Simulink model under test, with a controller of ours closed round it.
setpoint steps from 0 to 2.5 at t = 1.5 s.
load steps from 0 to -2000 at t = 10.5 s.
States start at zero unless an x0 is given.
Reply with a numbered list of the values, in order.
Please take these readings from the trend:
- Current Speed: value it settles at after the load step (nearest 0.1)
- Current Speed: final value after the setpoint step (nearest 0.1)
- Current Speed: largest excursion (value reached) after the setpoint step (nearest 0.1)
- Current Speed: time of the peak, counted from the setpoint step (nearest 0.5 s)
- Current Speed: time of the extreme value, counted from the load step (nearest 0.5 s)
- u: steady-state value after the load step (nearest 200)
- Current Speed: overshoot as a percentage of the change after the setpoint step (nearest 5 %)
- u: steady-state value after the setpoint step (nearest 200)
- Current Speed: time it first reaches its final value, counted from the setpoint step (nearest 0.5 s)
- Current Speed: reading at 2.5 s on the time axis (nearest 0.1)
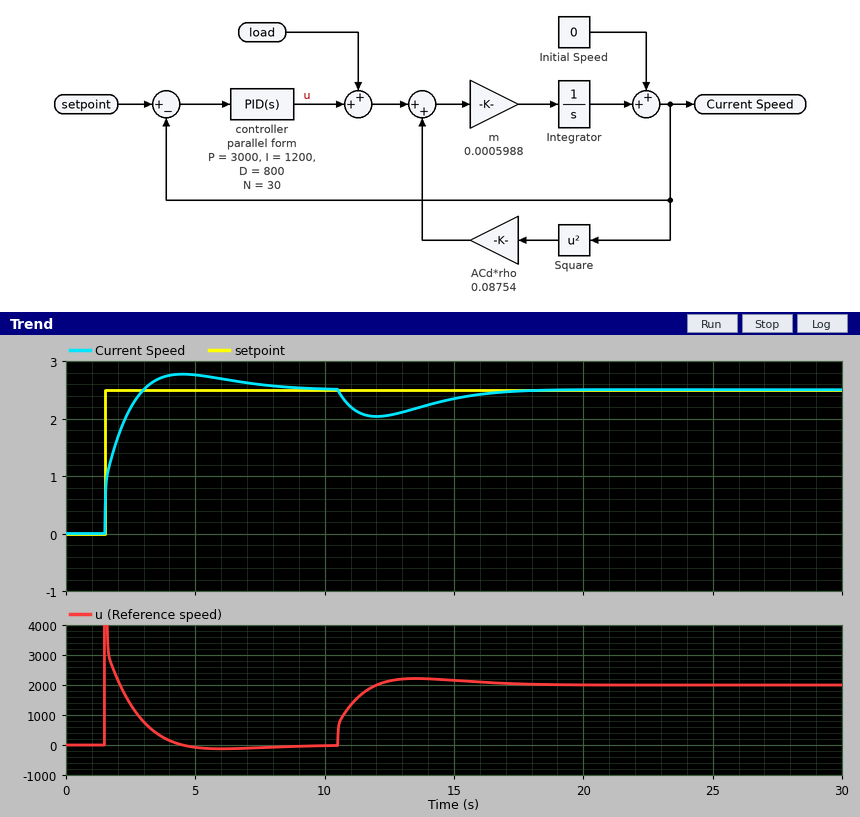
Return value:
1. 2.5
2. 2.5
3. 2.8
4. 3.0 s
5. 1.5 s
6. 2000
7. 10 %
8. 0
9. 1.5 s
10. 2.2
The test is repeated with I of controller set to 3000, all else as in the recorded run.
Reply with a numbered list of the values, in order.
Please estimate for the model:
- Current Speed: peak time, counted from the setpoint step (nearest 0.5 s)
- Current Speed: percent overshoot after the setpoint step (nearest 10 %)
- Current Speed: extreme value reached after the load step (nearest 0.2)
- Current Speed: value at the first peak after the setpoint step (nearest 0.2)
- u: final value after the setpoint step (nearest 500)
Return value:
1. 2.0 s
2. 20 %
3. 2.2
4. 3.0
5. 0
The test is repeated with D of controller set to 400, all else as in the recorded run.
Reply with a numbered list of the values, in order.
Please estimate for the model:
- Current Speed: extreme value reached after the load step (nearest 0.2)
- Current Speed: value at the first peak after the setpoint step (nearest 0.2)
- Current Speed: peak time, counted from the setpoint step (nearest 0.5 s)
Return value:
1. 2.0
2. 2.8
3. 2.5 s
